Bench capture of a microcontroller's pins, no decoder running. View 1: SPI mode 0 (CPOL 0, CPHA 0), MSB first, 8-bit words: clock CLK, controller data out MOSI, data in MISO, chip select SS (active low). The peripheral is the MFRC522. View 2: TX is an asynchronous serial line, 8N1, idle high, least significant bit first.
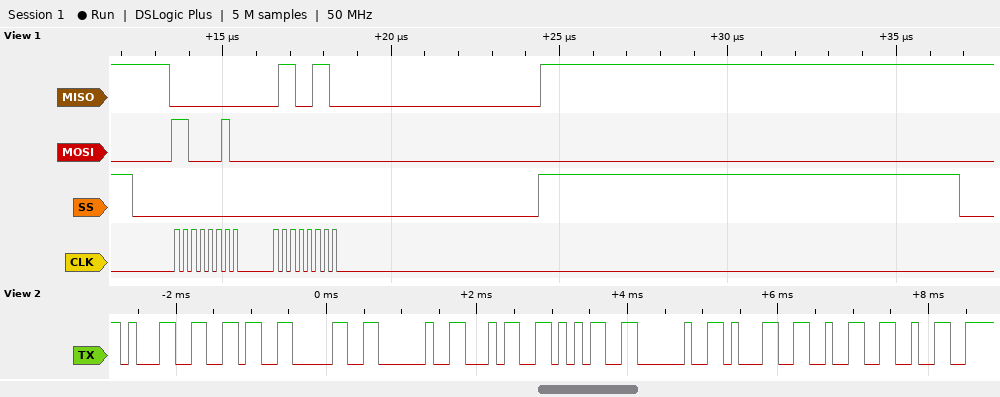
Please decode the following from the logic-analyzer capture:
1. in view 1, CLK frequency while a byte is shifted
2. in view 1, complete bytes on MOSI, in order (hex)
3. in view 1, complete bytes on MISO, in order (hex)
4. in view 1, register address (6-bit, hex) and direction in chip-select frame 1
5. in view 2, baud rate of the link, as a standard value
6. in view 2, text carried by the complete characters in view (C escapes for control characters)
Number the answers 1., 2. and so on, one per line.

1. 4 MHz
2. C2 00
3. 00 66
4. 0x21 read
5. 9600 baud
6. "160 45 122"
